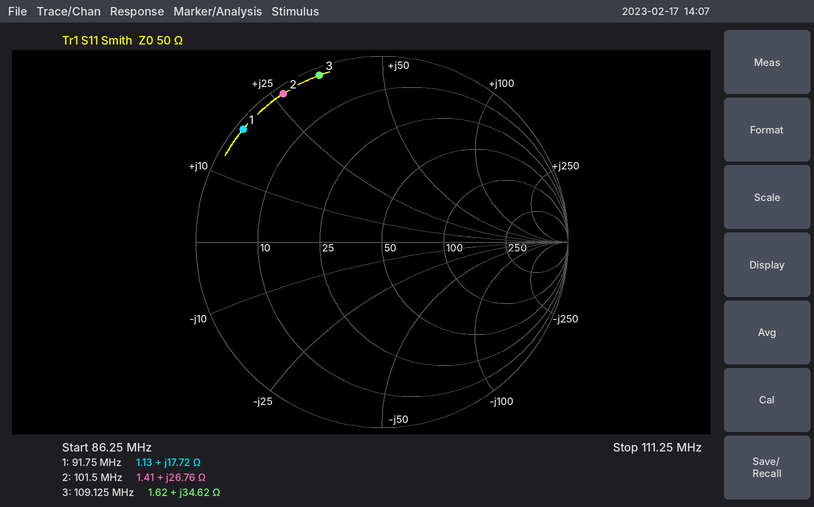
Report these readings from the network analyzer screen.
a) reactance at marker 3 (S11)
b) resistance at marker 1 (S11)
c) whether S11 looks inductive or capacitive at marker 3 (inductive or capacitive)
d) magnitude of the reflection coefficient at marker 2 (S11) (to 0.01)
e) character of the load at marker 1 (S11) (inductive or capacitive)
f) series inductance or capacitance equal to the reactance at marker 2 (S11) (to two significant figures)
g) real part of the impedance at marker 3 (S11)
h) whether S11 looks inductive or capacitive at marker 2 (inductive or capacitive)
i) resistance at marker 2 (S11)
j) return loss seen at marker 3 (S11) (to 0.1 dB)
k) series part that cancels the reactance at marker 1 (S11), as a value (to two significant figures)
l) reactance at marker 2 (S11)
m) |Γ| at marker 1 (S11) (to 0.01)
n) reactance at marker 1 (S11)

+34.62 Ω
1.13 Ω
inductive
0.96
inductive
42 nH
1.62 Ω
inductive
1.41 Ω
0.4 dB
98 pF
+26.76 Ω
0.96
+17.72 Ω
